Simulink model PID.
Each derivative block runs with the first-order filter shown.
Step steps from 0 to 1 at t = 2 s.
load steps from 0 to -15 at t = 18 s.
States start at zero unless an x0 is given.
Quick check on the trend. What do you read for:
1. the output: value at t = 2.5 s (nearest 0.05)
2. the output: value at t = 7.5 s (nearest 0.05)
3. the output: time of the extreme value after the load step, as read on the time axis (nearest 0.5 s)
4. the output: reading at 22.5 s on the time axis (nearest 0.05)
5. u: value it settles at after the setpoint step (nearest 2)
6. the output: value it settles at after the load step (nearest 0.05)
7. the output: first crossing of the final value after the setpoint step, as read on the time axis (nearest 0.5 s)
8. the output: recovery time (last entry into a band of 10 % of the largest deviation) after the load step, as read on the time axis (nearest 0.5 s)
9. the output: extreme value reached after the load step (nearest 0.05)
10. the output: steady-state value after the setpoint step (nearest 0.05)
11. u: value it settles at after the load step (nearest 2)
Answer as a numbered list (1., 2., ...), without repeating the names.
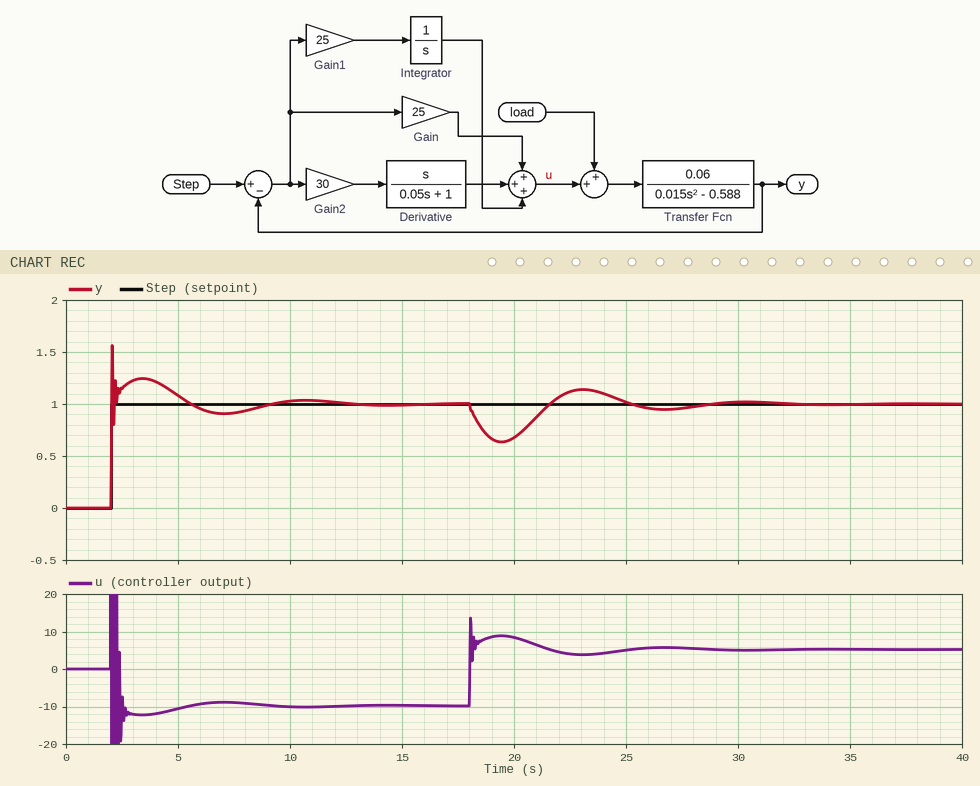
1. 1.15
2. 0.90
3. 19.5 s
4. 1.10
5. -10
6. 1.00
7. 2.0 s
8. 27.5 s
9. 0.65
10. 1.00
11. 6
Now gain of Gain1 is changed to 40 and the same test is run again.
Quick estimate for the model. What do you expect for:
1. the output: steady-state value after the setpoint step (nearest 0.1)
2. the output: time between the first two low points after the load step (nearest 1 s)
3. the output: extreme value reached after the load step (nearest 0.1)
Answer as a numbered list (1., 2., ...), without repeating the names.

1. 1.0
2. 6 s
3. 0.7
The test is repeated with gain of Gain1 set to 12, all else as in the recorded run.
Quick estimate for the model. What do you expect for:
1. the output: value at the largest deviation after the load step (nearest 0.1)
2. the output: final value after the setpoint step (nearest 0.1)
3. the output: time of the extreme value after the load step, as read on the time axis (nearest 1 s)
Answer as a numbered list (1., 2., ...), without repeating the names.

1. 0.5
2. 1.0
3. 20 s
